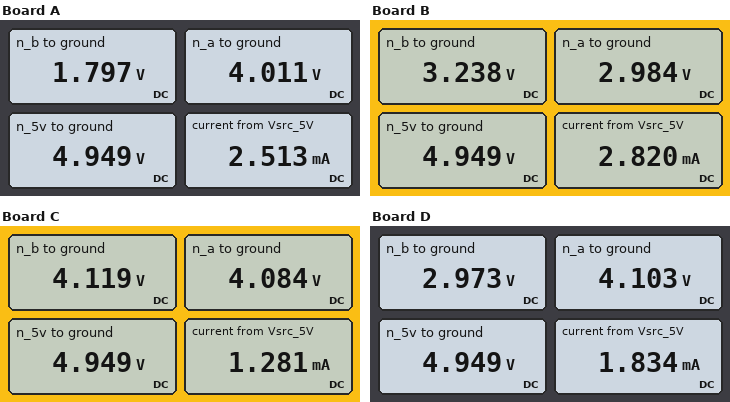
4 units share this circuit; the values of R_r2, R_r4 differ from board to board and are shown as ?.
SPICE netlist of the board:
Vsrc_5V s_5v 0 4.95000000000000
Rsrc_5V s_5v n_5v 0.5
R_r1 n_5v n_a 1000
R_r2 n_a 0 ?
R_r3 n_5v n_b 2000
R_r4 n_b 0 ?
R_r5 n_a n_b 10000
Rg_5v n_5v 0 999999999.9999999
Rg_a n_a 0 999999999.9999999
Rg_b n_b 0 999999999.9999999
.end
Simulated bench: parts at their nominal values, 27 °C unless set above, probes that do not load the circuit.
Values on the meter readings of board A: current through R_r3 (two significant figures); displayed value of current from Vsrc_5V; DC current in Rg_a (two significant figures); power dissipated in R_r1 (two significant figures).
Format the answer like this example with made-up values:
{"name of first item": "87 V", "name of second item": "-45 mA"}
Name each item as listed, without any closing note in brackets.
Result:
{"current through R_r3": "1.6 mA", "displayed value of current from Vsrc_5V": "2.513 mA", "DC current in Rg_a": "4.0 nA", "power dissipated in R_r1": "880 µW"}
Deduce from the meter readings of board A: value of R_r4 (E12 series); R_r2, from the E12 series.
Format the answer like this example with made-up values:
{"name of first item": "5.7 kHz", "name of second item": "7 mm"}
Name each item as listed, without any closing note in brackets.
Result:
{"value of R_r4": "1 kΩ", "R_r2, from the E12 series": "5.6 kΩ"}
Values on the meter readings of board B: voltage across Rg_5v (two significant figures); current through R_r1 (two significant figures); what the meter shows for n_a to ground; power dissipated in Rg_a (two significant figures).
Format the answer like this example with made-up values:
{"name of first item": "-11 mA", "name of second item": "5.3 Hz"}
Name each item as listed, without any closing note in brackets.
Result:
{"voltage across Rg_5v": "4.9 V", "current through R_r1": "2.0 mA", "what the meter shows for n_a to ground": "2.984 V", "power dissipated in Rg_a": "8.9 nW"}
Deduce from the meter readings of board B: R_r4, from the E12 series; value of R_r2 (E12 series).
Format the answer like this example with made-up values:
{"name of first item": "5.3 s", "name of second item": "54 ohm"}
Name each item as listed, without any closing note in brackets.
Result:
{"R_r4, from the E12 series": "3.9 kΩ", "value of R_r2": "1.5 kΩ"}
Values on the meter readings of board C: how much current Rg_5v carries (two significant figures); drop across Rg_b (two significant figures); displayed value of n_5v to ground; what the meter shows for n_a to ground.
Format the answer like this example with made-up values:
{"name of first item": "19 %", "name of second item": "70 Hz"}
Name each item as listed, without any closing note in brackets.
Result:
{"how much current Rg_5v carries": "4.9 nA", "drop across Rg_b": "4.1 V", "displayed value of n_5v to ground": "4.949 V", "what the meter shows for n_a to ground": "4.084 V"}
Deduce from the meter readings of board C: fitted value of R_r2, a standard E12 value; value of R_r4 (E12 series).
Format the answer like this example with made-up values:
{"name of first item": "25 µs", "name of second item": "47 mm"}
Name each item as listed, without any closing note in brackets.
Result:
{"fitted value of R_r2, a standard E12 value": "4.7 kΩ", "value of R_r4": "10 kΩ"}
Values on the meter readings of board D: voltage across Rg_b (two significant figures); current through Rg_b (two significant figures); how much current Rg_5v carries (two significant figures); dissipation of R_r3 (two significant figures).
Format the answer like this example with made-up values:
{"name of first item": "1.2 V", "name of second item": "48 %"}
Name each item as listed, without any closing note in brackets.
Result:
{"voltage across Rg_b": "3.0 V", "current through Rg_b": "3.0 nA", "how much current Rg_5v carries": "4.9 nA", "dissipation of R_r3": "2.0 mW"}
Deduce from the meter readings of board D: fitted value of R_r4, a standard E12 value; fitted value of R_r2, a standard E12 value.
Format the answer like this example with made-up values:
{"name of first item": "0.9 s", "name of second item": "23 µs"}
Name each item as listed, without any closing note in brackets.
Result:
{"fitted value of R_r4, a standard E12 value": "2.7 kΩ", "fitted value of R_r2, a standard E12 value": "5.6 kΩ"}
